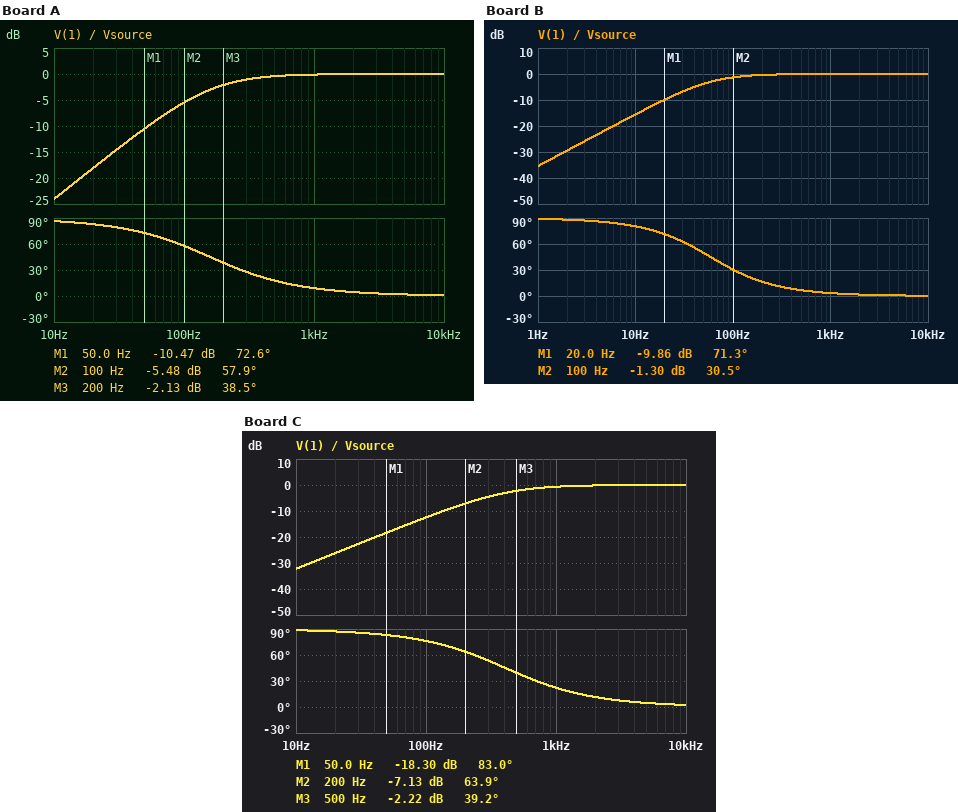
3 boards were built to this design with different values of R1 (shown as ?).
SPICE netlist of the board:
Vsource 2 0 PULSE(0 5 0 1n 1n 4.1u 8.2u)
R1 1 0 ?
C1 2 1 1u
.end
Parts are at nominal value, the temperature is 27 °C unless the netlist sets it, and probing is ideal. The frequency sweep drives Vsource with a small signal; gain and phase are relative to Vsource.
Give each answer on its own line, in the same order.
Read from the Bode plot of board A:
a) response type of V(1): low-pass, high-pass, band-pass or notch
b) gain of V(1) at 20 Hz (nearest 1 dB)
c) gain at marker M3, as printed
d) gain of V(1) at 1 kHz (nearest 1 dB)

high-pass
-18 dB
-2.13 dB
0 dB
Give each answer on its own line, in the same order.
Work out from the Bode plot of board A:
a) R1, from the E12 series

1 kΩ
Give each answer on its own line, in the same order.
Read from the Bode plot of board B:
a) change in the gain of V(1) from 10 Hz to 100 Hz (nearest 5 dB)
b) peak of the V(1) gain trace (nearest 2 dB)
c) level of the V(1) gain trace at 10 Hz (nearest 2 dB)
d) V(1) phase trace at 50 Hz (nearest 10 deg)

15 dB
0 dB
-16 dB
50 deg
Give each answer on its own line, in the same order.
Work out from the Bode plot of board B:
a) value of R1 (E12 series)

2.7 kΩ
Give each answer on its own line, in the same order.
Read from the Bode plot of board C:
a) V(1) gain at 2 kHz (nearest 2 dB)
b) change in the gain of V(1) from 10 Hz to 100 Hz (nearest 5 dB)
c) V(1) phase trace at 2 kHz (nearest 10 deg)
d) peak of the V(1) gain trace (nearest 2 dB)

0 dB
20 dB
10 deg
0 dB
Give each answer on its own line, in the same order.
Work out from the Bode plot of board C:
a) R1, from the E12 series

390 Ω
